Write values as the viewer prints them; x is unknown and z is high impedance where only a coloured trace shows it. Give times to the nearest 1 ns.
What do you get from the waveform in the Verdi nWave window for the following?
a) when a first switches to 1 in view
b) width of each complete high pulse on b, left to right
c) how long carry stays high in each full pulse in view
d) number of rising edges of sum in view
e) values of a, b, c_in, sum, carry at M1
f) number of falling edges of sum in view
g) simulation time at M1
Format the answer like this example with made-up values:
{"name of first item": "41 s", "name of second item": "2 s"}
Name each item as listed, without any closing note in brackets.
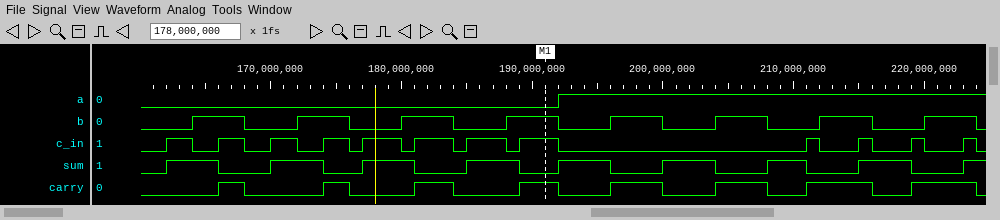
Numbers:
{"when a first switches to 1 in view": "192 ns", "width of each complete high pulse on b, left to right": "4 ns, 4 ns, 4 ns, 4 ns, 4 ns, 4 ns, 4 ns, 4 ns", "how long carry stays high in each full pulse in view": "2 ns, 2 ns, 3 ns, 3 ns, 4 ns, 4 ns, 5 ns, 5 ns", "number of rising edges of sum in view": "9", "values of a, b, c_in, sum, carry at M1": "a=0, b=1, c_in=1, sum=0, carry=1", "number of falling edges of sum in view": "8", "simulation time at M1": "191 ns"}
